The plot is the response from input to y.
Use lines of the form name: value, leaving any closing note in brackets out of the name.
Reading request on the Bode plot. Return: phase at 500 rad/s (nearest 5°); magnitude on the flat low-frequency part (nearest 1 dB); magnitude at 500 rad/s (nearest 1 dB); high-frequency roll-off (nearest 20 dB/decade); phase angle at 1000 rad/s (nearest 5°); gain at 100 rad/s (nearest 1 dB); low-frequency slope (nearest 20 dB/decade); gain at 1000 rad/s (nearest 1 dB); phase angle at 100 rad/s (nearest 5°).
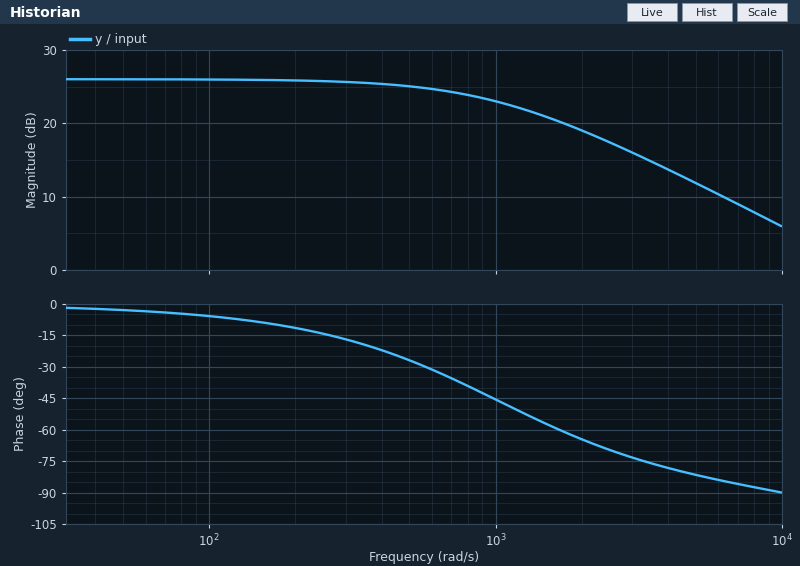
phase at 500 rad/s: -25°
magnitude on the flat low-frequency part: 26 dB
magnitude at 500 rad/s: 25 dB
high-frequency roll-off: -20 dB/decade
phase angle at 1000 rad/s: -45°
gain at 100 rad/s: 26 dB
low-frequency slope: 0 dB/decade
gain at 1000 rad/s: 23 dB
phase angle at 100 rad/s: -5°
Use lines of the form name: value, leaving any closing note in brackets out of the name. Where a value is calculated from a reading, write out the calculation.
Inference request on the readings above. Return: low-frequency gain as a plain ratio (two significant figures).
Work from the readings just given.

low-frequency gain as a plain ratio: 10^(26 / 20) = 20
